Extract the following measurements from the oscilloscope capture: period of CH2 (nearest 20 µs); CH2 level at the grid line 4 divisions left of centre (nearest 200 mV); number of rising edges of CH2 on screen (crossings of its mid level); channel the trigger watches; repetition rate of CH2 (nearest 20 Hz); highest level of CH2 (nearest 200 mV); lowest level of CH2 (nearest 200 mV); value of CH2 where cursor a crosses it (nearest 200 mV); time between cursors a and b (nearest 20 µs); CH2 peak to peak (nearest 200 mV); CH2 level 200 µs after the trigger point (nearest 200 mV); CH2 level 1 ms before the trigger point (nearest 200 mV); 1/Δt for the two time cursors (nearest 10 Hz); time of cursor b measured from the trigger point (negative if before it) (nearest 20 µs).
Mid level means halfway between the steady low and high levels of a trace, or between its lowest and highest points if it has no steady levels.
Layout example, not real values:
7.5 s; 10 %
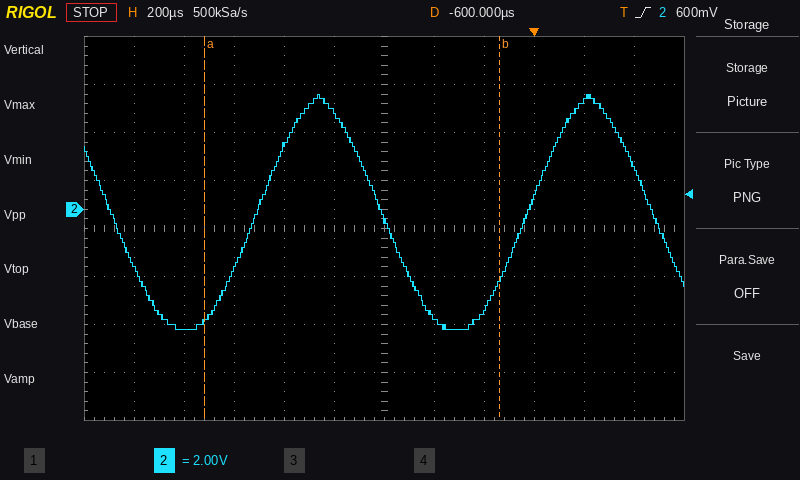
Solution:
1.08 ms; -5.0 V; 2; CH2; 920 Hz; 4.8 V; -5.0 V; -4.6 V; 1.18 ms; 9.8 V; 4.6 V; 2.6 V; 850 Hz; -140 µs
